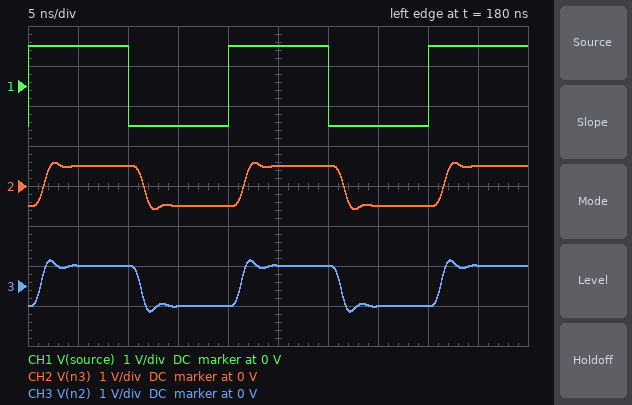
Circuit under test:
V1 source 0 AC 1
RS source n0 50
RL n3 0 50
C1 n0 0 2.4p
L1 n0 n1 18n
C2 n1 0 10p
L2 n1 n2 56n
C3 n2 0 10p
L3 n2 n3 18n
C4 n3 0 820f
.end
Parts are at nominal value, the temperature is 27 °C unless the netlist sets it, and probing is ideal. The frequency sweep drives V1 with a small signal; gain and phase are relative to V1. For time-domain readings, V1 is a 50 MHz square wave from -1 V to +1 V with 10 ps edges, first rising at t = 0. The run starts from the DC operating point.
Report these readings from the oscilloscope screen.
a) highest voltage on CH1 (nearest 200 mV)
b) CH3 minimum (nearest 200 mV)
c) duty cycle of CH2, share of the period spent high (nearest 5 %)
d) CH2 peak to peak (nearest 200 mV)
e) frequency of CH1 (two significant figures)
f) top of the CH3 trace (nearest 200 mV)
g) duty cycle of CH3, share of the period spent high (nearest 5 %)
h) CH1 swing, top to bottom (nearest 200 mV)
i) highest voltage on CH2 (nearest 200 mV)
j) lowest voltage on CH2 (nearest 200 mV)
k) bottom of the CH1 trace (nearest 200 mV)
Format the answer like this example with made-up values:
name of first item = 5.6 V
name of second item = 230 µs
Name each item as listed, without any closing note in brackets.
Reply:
highest voltage on CH1 = 1.0 V
CH3 minimum = -600 mV
duty cycle of CH2, share of the period spent high = 50 %
CH2 peak to peak = 1.2 V
frequency of CH1 = 50 MHz
top of the CH3 trace = 600 mV
duty cycle of CH3, share of the period spent high = 50 %
CH1 swing, top to bottom = 2.0 V
highest voltage on CH2 = 600 mV
lowest voltage on CH2 = -600 mV
bottom of the CH1 trace = -1.0 V
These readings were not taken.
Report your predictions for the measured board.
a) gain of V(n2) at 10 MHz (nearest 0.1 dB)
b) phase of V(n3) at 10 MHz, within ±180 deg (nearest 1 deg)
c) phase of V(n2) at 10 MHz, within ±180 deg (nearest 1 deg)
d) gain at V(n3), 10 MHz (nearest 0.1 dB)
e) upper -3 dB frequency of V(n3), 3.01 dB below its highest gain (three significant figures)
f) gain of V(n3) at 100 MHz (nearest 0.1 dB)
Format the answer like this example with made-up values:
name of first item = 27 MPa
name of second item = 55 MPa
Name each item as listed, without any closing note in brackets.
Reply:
gain of V(n2) at 10 MHz = -6.0 dB
phase of V(n3) at 10 MHz, within ±180 deg = -5 deg
phase of V(n2) at 10 MHz, within ±180 deg = -4 deg
gain at V(n3), 10 MHz = -6.0 dB
upper -3 dB frequency of V(n3), 3.01 dB below its highest gain = 397 MHz
gain of V(n3) at 100 MHz = -6.2 dB
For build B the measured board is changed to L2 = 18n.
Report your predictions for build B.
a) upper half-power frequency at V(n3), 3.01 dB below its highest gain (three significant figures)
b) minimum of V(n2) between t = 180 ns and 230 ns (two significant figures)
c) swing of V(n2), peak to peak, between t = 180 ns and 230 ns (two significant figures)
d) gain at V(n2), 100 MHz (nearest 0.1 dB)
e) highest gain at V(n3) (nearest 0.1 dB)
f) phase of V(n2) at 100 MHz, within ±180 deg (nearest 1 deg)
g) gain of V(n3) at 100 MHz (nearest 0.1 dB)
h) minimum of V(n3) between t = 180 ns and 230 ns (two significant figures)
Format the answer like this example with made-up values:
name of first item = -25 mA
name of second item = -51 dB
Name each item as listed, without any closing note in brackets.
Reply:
upper half-power frequency at V(n3), 3.01 dB below its highest gain = 667 MHz
minimum of V(n2) between t = 180 ns and 230 ns = -780 mV
swing of V(n2), peak to peak, between t = 180 ns and 230 ns = 1.6 V
gain at V(n2), 100 MHz = -5.9 dB
highest gain at V(n3) = -6.0 dB
phase of V(n2) at 100 MHz, within ±180 deg = -28 deg
gain of V(n3) at 100 MHz = -6.0 dB
minimum of V(n3) between t = 180 ns and 230 ns = -640 mV
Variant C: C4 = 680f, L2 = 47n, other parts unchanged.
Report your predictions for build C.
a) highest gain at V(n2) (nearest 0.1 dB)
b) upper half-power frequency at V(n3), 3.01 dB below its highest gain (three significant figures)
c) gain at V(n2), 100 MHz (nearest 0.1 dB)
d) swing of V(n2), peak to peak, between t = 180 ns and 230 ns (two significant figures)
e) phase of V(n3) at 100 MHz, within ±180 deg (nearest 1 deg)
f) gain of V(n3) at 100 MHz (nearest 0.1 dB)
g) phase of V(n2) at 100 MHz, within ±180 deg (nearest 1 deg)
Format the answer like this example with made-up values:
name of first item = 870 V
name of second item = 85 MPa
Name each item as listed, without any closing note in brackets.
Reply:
highest gain at V(n2) = -5.0 dB
upper half-power frequency at V(n3), 3.01 dB below its highest gain = 441 MHz
gain at V(n2), 100 MHz = -5.9 dB
swing of V(n2), peak to peak, between t = 180 ns and 230 ns = 1.4 V
phase of V(n3) at 100 MHz, within ±180 deg = -51 deg
gain of V(n3) at 100 MHz = -6.1 dB
phase of V(n2) at 100 MHz, within ±180 deg = -38 deg
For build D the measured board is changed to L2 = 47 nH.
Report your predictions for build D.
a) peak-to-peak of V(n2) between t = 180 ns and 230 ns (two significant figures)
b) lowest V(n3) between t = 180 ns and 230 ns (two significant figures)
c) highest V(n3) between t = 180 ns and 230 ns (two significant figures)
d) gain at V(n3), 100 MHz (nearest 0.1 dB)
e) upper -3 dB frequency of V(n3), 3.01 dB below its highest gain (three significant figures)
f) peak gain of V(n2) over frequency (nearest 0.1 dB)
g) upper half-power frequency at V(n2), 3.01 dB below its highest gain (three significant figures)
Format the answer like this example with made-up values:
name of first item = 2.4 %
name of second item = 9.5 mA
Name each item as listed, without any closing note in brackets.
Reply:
peak-to-peak of V(n2) between t = 180 ns and 230 ns = 1.4 V
lowest V(n3) between t = 180 ns and 230 ns = -610 mV
highest V(n3) between t = 180 ns and 230 ns = 610 mV
gain at V(n3), 100 MHz = -6.1 dB
upper -3 dB frequency of V(n3), 3.01 dB below its highest gain = 441 MHz
peak gain of V(n2) over frequency = -5.1 dB
upper half-power frequency at V(n2), 3.01 dB below its highest gain = 478 MHz
